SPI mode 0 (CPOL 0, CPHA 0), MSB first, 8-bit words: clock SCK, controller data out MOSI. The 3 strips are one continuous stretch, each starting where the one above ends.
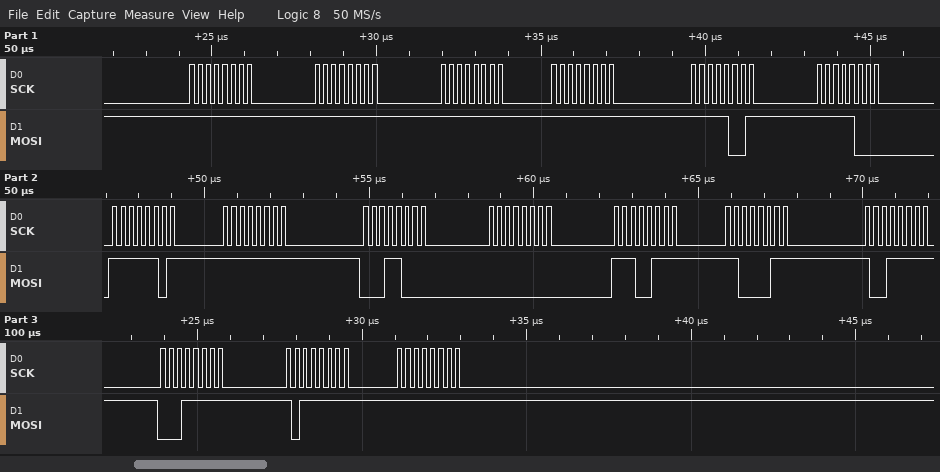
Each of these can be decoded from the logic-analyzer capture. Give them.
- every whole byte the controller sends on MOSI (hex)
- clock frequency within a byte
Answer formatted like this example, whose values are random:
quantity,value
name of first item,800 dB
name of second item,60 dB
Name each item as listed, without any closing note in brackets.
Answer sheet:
quantity,value
every whole byte the controller sends on MOSI,FF FF FF FF F9 F8 FD FF 18 00 E7 C3 9F 1F BF FF
clock frequency within a byte,4 MHz
